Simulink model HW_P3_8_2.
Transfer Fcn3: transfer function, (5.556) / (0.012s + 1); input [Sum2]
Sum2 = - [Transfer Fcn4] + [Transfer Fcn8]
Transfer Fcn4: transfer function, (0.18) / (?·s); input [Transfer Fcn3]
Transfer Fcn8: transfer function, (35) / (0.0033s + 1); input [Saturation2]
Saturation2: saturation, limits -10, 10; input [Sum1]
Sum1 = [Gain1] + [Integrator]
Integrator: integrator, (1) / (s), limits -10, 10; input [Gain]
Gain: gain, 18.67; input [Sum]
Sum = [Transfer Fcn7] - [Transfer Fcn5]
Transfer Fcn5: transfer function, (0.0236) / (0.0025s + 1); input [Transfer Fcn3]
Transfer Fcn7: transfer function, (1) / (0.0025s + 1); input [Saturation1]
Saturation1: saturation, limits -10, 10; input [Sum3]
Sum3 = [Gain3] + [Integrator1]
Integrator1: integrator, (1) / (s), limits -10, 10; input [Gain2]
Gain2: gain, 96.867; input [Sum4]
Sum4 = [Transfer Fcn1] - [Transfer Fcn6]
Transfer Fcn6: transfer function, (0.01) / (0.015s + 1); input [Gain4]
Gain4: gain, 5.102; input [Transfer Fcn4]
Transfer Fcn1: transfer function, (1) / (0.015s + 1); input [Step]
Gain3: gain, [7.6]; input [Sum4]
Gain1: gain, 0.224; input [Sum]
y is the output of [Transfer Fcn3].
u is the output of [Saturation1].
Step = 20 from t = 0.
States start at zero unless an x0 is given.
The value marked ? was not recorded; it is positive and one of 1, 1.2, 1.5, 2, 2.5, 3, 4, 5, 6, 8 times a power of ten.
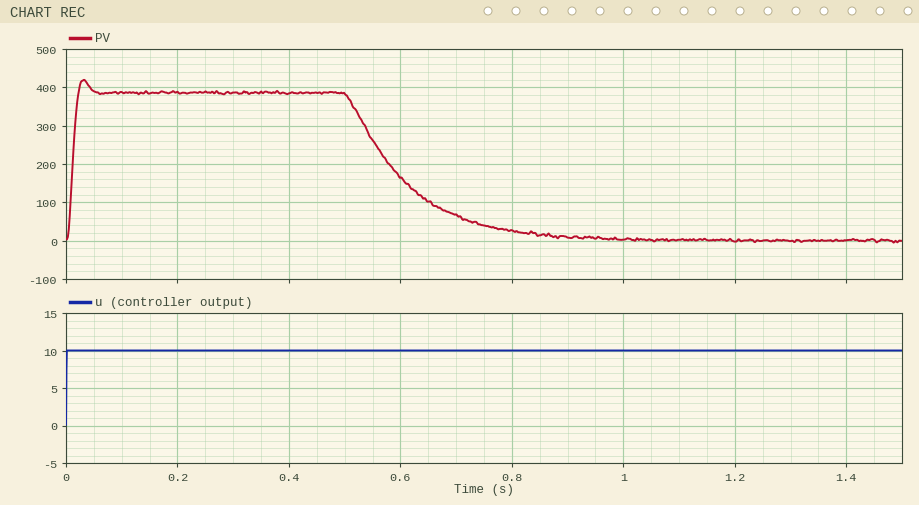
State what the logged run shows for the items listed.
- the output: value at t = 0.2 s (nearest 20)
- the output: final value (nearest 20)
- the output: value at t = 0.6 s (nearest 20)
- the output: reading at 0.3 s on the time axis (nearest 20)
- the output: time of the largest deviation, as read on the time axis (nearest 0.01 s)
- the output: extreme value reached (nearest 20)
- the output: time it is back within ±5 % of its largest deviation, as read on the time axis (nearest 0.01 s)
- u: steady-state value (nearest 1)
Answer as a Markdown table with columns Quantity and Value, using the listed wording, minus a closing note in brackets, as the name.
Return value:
| Quantity | Value |
|---|---|
| the output: value at t = 0.2 s | 380 |
| the output: final value | 0 |
| the output: value at t = 0.6 s | 160 |
| the output: reading at 0.3 s on the time axis | 380 |
| the output: time of the largest deviation, as read on the time axis | 0.03 s |
| the output: extreme value reached | 420 |
| the output: time it is back within ±5 % of its largest deviation, as read on the time axis | 0.82 s |
| u: steady-state value | 10 |
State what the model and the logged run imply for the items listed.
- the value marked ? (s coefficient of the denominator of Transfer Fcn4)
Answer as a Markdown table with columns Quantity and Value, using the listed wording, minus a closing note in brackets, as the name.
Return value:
| Quantity | Value |
|---|---|
| the value marked ? | 0.12 |
